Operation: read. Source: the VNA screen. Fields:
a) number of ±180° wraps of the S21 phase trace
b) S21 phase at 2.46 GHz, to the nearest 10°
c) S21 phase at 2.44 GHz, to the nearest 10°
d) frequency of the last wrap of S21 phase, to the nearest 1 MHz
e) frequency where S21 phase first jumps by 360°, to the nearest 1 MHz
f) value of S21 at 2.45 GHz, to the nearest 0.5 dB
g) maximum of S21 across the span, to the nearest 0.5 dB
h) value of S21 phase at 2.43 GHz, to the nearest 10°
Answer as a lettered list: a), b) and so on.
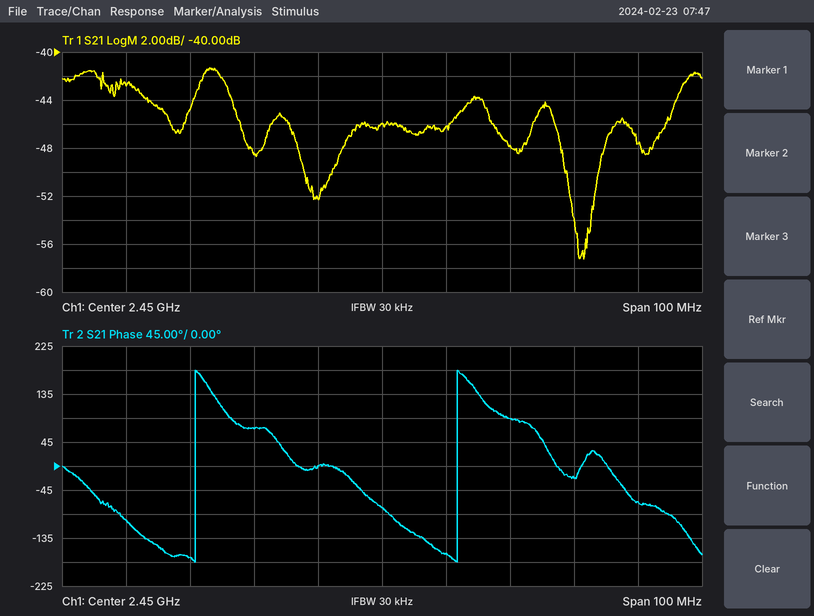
a) 2
b) -160°
c) 0°
d) 2.462 GHz
e) 2.421 GHz
f) -46.0 dB
g) -41.5 dB
h) 70°
